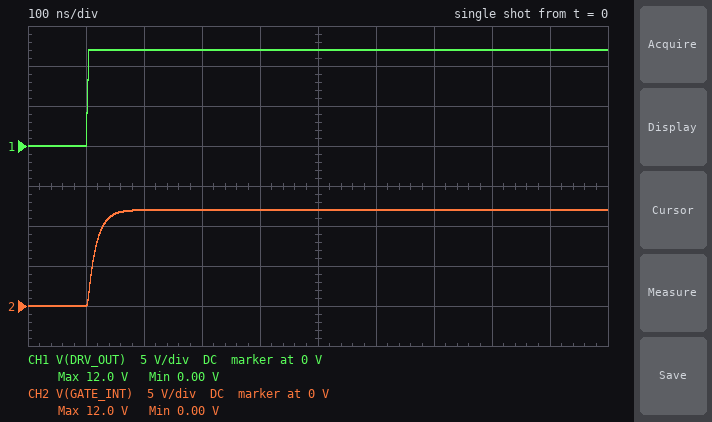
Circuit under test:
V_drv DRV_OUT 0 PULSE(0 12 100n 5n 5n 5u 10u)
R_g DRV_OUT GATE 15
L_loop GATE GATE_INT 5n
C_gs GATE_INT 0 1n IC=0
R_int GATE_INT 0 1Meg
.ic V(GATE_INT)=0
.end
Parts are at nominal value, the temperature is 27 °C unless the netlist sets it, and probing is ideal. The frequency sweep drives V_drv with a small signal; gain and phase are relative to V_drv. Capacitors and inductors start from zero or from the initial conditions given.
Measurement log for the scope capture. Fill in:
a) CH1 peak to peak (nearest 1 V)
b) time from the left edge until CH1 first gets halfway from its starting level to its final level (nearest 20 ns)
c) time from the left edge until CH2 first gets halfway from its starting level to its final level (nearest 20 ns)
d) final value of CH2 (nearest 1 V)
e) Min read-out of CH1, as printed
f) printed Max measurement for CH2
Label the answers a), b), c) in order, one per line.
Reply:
a) 12 V
b) 100 ns
c) 120 ns
d) 12 V
e) 0.00 V
f) 12.0 V
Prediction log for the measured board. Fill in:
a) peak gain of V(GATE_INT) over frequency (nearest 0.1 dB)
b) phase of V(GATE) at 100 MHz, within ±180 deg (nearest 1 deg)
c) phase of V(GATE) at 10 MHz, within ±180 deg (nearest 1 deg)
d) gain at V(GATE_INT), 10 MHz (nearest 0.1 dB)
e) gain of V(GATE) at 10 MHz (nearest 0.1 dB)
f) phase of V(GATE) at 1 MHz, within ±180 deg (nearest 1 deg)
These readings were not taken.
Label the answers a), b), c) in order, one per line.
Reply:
a) 0 dB
b) 84 deg
c) -44 deg
d) -2.7 dB
e) -2.8 dB
f) -5 deg
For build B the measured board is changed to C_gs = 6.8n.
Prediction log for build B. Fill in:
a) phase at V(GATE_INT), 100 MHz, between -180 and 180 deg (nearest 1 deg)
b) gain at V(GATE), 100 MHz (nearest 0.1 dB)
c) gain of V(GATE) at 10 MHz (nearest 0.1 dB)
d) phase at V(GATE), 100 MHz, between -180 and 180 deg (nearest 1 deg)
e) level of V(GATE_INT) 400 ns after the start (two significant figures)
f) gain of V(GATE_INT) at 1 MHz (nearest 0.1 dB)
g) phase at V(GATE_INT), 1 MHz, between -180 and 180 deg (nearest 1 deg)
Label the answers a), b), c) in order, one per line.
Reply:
a) -101 deg
b) -14.4 dB
c) -17.5 dB
d) 79 deg
e) 11 V
f) -1.5 dB
g) -33 deg
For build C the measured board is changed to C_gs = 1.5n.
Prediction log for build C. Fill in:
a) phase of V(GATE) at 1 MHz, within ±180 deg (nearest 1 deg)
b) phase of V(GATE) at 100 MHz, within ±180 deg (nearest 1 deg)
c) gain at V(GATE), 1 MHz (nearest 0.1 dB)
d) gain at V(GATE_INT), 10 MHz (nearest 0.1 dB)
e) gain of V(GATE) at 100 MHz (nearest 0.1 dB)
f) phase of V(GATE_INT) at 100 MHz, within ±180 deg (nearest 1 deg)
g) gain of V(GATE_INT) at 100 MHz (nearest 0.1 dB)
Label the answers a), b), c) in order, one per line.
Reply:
a) -8 deg
b) 82 deg
c) -0.1 dB
d) -4.7 dB
e) -17.2 dB
f) -98 deg
g) -23.1 dB
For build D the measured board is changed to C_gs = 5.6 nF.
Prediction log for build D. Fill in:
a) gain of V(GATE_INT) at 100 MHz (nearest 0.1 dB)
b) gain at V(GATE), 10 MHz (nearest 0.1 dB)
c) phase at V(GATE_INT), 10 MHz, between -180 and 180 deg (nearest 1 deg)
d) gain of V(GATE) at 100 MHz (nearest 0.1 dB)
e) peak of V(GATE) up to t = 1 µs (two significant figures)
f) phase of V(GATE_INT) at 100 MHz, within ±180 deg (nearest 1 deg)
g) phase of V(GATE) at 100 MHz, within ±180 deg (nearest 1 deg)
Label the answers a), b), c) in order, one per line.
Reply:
a) -34.6 dB
b) -15.6 dB
c) -80 deg
d) -14.6 dB
e) 12 V
f) -101 deg
g) 79 deg
